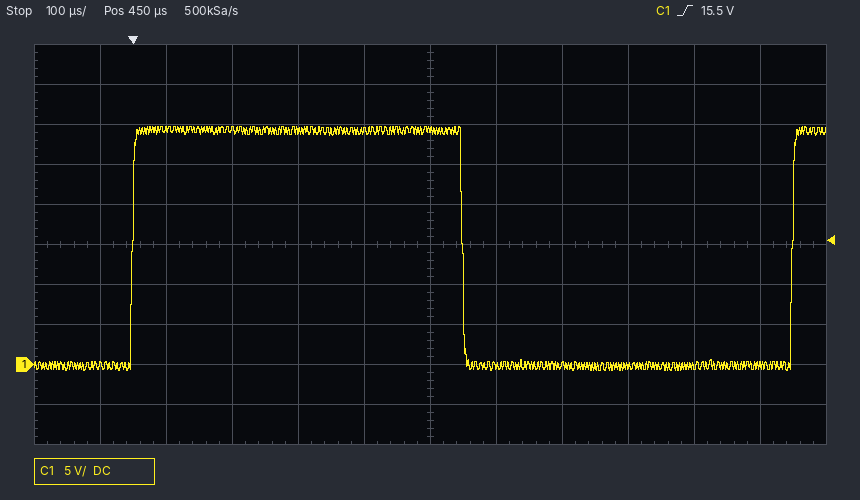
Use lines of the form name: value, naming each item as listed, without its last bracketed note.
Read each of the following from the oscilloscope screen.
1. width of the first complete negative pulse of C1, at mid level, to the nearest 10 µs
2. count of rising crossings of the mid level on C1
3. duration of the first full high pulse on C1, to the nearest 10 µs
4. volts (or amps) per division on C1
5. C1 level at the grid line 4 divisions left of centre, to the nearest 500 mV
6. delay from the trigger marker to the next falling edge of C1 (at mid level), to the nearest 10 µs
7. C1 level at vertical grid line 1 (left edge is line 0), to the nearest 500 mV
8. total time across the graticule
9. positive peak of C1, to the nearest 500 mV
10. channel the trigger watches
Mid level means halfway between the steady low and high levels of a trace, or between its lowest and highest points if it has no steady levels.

width of the first complete negative pulse of C1, at mid level, to the nearest 10 µs: 500 µs
count of rising crossings of the mid level on C1: 2
duration of the first full high pulse on C1, to the nearest 10 µs: 500 µs
volts (or amps) per division on C1: 5 V
C1 level at the grid line 4 divisions left of centre, to the nearest 500 mV: 29.5 V
delay from the trigger marker to the next falling edge of C1 (at mid level), to the nearest 10 µs: 500 µs
C1 level at vertical grid line 1 (left edge is line 0), to the nearest 500 mV: 0.0 V
total time across the graticule: 1.2 ms
positive peak of C1, to the nearest 500 mV: 30.0 V
channel the trigger watches: C1
